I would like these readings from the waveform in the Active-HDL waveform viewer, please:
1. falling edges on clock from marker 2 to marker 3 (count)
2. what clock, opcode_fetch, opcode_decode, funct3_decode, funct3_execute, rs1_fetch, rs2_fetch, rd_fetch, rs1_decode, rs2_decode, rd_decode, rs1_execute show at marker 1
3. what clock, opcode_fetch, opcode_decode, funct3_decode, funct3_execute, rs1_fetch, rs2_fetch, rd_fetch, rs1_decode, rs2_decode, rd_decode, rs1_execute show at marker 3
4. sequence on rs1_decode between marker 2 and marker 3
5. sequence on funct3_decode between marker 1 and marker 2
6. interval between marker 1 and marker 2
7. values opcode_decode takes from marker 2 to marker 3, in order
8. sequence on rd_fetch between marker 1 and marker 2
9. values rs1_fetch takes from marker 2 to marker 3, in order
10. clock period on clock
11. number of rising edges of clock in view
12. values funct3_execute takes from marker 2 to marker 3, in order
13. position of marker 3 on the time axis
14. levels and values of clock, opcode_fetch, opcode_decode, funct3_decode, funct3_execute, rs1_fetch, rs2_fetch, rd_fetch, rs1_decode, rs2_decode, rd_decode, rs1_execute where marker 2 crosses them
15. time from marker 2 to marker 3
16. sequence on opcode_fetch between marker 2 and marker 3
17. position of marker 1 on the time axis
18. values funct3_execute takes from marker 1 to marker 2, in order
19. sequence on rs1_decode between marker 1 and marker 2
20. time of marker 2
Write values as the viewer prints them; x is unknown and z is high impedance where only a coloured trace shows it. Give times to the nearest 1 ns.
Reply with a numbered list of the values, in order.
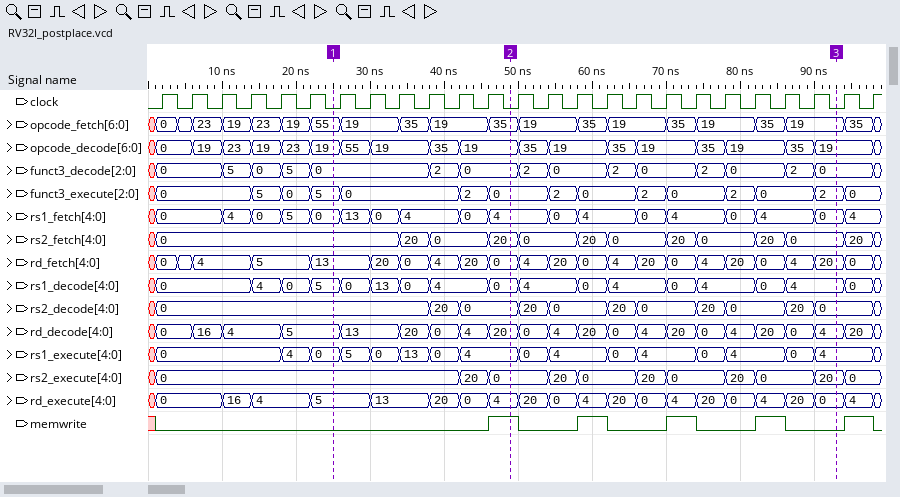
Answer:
1. 11
2. clock=0, opcode_fetch=55, opcode_decode=19, funct3_decode=0, funct3_execute=5, rs1_fetch=0, rs2_fetch=0, rd_fetch=13, rs1_decode=5, rs2_decode=0, rd_decode=5, rs1_execute=0
3. clock=0, opcode_fetch=19, opcode_decode=19, funct3_decode=0, funct3_execute=2, rs1_fetch=0, rs2_fetch=0, rd_fetch=20, rs1_decode=4, rs2_decode=0, rd_decode=4, rs1_execute=4
4. 0, 4, 0, 4, 0, 4, 0, 4
5. 0, 2, 0
6. 24 ns
7. 19, 35, 19, 35, 19, 35, 19, 35, 19
8. 13, 20, 0, 4, 20, 0
9. 4, 0, 4, 0, 4, 0, 4, 0
10. 4 ns
11. 25
12. 0, 2, 0, 2, 0, 2, 0, 2
13. 93 ns
14. clock=0, opcode_fetch=35, opcode_decode=19, funct3_decode=0, funct3_execute=0, rs1_fetch=4, rs2_fetch=20, rd_fetch=0, rs1_decode=0, rs2_decode=0, rd_decode=20, rs1_execute=4
15. 44 ns
16. 35, 19, 35, 19, 35, 19, 35, 19
17. 25 ns
18. 5, 0, 2, 0
19. 5, 0, 13, 0, 4, 0
20. 49 ns
